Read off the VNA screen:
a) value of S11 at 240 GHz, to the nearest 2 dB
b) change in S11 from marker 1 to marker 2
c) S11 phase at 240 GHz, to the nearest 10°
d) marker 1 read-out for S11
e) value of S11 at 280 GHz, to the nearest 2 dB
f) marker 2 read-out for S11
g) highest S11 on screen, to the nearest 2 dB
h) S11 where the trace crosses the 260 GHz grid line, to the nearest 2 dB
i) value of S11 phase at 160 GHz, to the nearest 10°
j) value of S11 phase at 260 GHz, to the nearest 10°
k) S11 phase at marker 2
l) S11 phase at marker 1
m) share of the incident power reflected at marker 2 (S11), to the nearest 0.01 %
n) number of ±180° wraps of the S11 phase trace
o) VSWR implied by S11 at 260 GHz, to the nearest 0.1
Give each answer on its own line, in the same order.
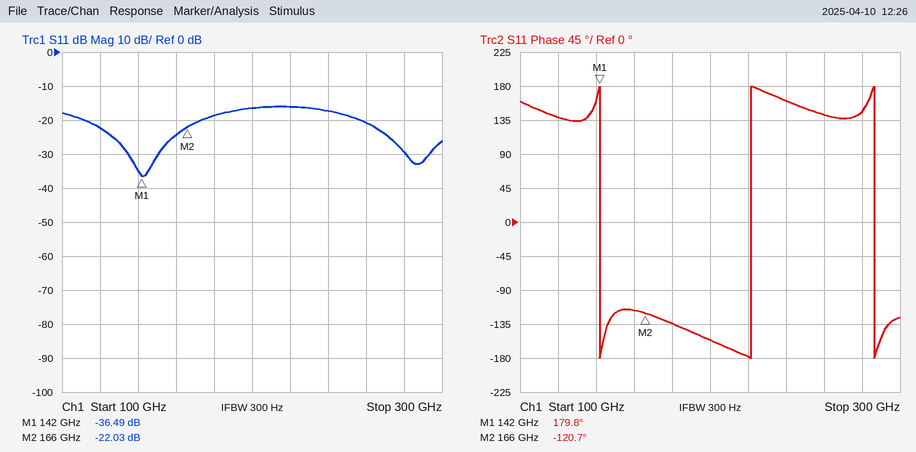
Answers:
-18 dB
14.46 dB
160°
-36.49 dB
-30 dB
-22.03 dB
-16 dB
-20 dB
-120°
140°
-120.7°
179.8°
0.63 %
3
1.2
